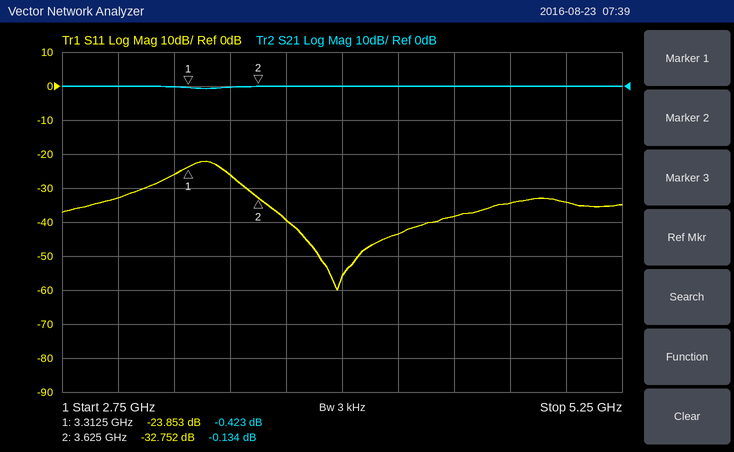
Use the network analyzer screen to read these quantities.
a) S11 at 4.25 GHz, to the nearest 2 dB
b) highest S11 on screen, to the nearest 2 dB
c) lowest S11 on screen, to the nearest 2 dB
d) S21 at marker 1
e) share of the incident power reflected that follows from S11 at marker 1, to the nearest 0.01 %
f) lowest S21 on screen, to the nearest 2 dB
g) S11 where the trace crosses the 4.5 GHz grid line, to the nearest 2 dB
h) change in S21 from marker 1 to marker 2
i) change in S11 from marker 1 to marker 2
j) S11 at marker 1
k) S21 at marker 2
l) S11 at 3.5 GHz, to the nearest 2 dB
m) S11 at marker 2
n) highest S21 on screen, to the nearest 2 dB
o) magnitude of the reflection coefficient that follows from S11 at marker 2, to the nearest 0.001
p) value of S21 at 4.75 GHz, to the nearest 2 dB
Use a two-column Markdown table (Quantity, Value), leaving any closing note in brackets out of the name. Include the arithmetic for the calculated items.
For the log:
| Quantity | Value |
|---|---|
| S11 at 4.25 GHz, to the nearest 2 dB | -44 dB |
| highest S11 on screen, to the nearest 2 dB | -22 dB |
| lowest S11 on screen, to the nearest 2 dB | -60 dB |
| S21 at marker 1 | -0.423 dB |
| share of the incident power reflected that follows from S11 at marker 1, to the nearest 0.01 % | 10^(-23.853/10) ≈ 0.41 % |
| lowest S21 on screen, to the nearest 2 dB | 0 dB |
| S11 where the trace crosses the 4.5 GHz grid line, to the nearest 2 dB | -38 dB |
| change in S21 from marker 1 to marker 2 | -0.134 − (-0.423) = 0.289 dB |
| change in S11 from marker 1 to marker 2 | -32.752 − (-23.853) = -8.899 dB |
| S11 at marker 1 | -23.853 dB |
| S21 at marker 2 | -0.134 dB |
| S11 at 3.5 GHz, to the nearest 2 dB | -26 dB |
| S11 at marker 2 | -32.752 dB |
| highest S21 on screen, to the nearest 2 dB | 0 dB |
| magnitude of the reflection coefficient that follows from S11 at marker 2, to the nearest 0.001 | 10^(-32.752/20) ≈ 0.023 |
| value of S21 at 4.75 GHz, to the nearest 2 dB | 0 dB |
